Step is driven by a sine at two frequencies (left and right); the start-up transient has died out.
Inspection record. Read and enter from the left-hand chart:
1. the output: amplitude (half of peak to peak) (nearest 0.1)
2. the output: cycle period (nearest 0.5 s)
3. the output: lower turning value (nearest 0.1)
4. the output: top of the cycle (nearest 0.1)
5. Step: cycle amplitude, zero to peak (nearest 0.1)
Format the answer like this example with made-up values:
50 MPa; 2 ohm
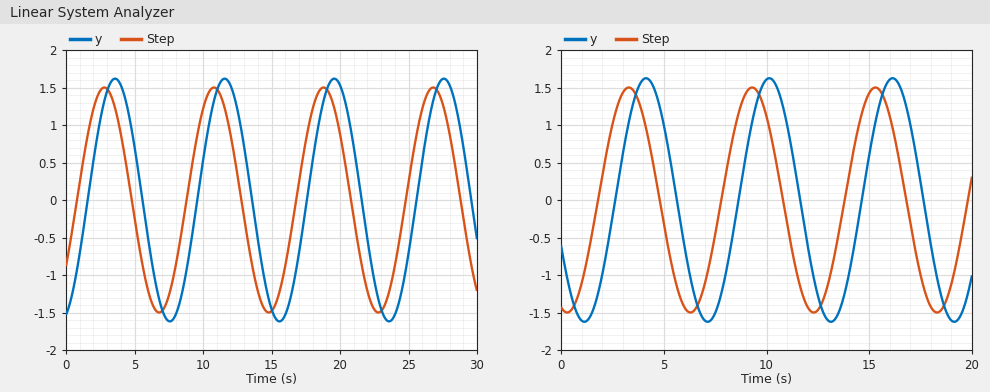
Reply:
1.6; 8.0 s; -1.6; 1.6; 1.5
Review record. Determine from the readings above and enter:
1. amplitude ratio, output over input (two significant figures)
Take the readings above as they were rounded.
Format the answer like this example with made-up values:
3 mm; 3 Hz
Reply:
1.1
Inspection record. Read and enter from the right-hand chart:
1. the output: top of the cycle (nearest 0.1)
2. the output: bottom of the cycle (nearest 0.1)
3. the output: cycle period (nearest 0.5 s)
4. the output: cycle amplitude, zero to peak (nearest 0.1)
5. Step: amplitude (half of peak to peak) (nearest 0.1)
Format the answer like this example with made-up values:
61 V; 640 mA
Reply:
1.6; -1.6; 6.0 s; 1.6; 1.5
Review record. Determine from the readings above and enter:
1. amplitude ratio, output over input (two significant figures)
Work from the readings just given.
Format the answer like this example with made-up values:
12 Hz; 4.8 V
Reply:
1.1
